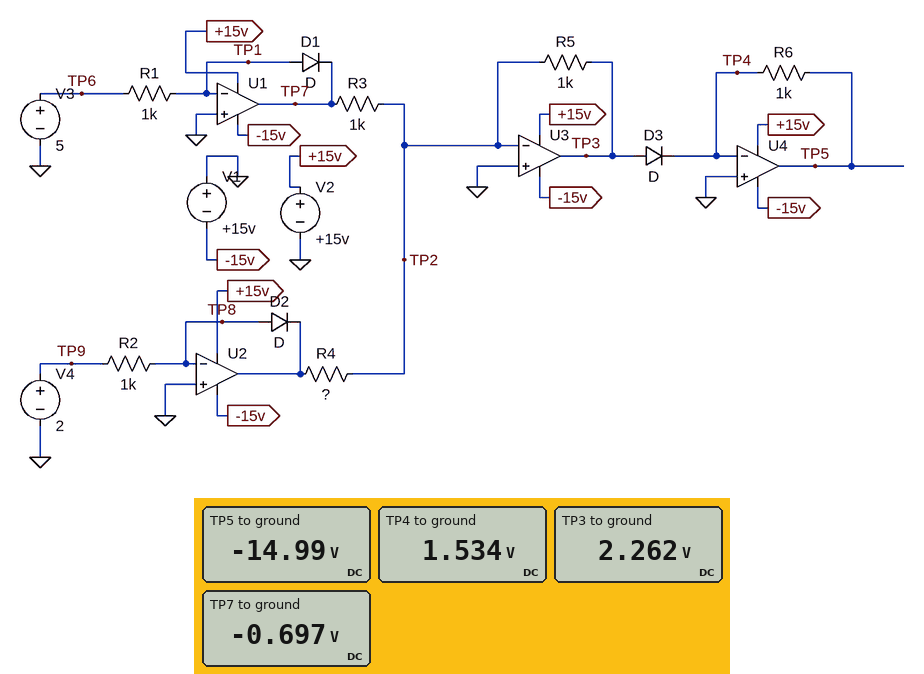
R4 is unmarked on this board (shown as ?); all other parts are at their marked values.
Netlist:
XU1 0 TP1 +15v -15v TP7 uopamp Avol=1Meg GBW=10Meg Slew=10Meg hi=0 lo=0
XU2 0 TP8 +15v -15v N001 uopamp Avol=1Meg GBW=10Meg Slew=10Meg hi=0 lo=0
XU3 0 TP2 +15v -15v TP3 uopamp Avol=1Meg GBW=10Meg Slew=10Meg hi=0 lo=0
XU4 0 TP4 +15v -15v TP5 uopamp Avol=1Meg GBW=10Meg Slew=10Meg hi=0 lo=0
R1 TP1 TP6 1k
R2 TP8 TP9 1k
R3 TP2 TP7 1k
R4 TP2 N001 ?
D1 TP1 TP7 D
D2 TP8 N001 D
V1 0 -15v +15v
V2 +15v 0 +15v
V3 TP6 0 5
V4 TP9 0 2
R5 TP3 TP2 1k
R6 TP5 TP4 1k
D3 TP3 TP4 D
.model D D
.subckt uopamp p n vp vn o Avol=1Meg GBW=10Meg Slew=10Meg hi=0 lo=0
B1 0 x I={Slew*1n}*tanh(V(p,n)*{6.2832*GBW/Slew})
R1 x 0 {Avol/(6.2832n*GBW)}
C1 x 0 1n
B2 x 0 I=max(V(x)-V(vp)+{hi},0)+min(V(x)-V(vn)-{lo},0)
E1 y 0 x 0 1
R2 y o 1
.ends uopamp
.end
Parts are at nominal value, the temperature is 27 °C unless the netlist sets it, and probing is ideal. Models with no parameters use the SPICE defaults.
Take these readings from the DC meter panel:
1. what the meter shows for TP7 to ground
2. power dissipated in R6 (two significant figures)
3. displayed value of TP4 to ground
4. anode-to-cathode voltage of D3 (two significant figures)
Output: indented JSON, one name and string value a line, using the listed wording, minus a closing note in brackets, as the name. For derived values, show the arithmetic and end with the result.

{
  "what the meter shows for TP7 to ground": "-0.697 V",
  "power dissipated in R6": "(1.534 V - (-14.99 V))^2 / 1 kΩ = 270 mW",
  "displayed value of TP4 to ground": "1.534 V",
  "anode-to-cathode voltage of D3": "2.262 V - 1.534 V = 730 mV"
}
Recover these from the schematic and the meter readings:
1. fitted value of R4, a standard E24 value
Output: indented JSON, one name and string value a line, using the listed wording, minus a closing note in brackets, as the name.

{
  "fitted value of R4, a standard E24 value": "430 Ω"
}
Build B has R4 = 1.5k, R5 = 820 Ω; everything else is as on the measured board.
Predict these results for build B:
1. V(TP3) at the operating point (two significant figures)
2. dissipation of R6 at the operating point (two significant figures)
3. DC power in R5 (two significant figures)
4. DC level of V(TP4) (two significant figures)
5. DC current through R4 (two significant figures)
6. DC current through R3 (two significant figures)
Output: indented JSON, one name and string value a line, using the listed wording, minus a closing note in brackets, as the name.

{
  "V(TP3) at the operating point": "940 mV",
  "dissipation of R6 at the operating point": "230 mW",
  "DC power in R5": "1.1 mW",
  "DC level of V(TP4)": "210 mV",
  "DC current through R4": "450 µA",
  "DC current through R3": "700 µA"
}
